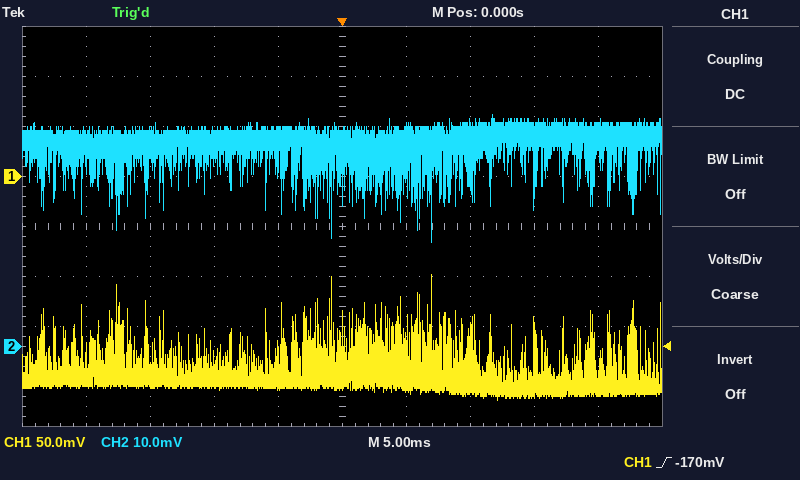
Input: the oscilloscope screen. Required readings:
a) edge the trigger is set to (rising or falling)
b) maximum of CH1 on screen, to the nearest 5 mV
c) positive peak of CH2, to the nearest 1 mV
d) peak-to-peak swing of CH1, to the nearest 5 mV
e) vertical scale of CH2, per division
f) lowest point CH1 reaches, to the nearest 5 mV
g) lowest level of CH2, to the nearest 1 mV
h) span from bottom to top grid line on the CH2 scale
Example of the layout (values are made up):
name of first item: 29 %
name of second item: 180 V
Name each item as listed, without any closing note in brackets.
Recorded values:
edge the trigger is set to: rising
maximum of CH1 on screen, to the nearest 5 mV: -100 mV
positive peak of CH2, to the nearest 1 mV: 46 mV
peak-to-peak swing of CH1, to the nearest 5 mV: 125 mV
vertical scale of CH2, per division: 10 mV
lowest point CH1 reaches, to the nearest 5 mV: -225 mV
lowest level of CH2, to the nearest 1 mV: 21 mV
span from bottom to top grid line on the CH2 scale: 80 mV
